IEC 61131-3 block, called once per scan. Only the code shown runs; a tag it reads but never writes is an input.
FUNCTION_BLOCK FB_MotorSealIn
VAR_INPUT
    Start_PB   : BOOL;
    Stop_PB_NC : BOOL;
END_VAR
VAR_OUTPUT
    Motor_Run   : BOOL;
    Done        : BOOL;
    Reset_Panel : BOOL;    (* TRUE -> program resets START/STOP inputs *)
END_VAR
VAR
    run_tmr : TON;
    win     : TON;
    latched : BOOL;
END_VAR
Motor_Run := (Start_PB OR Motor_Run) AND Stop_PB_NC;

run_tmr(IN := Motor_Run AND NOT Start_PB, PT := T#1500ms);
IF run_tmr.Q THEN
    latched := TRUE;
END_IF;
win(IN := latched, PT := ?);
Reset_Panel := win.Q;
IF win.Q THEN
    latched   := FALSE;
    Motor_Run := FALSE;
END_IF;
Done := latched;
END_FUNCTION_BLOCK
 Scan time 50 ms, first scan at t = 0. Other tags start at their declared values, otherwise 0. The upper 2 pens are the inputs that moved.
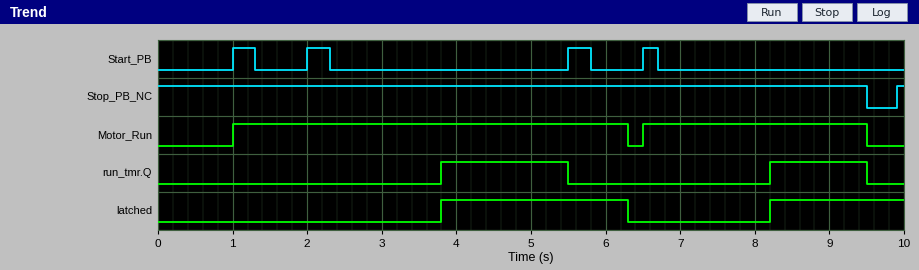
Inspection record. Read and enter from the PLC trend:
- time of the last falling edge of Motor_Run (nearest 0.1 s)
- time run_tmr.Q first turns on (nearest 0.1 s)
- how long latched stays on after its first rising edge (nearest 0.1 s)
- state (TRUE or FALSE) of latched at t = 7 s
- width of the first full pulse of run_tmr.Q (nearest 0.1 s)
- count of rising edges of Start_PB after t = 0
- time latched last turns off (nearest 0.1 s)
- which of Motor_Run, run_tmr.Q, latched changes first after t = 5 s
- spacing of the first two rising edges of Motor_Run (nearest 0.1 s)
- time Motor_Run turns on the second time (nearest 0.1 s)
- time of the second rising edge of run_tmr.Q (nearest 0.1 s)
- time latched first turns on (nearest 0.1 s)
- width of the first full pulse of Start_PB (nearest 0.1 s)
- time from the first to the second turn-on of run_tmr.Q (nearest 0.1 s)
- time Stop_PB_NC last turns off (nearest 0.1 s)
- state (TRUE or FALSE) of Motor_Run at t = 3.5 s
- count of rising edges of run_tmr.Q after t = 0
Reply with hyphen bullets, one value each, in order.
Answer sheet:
- 9.5 s
- 3.8 s
- 2.5 s
- FALSE
- 1.7 s
- 4
- 6.3 s
- run_tmr.Q
- 5.5 s
- 6.5 s
- 8.2 s
- 3.8 s
- 0.3 s
- 4.4 s
- 9.5 s
- TRUE
- 2
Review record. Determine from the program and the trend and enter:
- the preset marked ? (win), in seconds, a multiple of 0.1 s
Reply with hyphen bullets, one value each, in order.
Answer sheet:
- 2.5 s
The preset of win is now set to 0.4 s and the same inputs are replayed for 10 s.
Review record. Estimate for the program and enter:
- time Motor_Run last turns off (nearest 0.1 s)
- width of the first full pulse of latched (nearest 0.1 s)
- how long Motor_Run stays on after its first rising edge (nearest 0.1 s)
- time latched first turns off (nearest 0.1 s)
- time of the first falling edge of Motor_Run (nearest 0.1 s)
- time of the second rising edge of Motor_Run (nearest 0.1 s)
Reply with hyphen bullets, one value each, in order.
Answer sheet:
- 8.6 s
- 0.4 s
- 3.2 s
- 4.2 s
- 4.2 s
- 5.5 s
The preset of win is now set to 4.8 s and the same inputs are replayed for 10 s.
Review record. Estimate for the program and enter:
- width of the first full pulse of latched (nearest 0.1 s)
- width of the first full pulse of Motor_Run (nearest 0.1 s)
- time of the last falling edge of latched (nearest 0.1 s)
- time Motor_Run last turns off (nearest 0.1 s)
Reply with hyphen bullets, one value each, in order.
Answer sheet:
- 4.8 s
- 7.6 s
- 8.6 s
- 8.6 s
